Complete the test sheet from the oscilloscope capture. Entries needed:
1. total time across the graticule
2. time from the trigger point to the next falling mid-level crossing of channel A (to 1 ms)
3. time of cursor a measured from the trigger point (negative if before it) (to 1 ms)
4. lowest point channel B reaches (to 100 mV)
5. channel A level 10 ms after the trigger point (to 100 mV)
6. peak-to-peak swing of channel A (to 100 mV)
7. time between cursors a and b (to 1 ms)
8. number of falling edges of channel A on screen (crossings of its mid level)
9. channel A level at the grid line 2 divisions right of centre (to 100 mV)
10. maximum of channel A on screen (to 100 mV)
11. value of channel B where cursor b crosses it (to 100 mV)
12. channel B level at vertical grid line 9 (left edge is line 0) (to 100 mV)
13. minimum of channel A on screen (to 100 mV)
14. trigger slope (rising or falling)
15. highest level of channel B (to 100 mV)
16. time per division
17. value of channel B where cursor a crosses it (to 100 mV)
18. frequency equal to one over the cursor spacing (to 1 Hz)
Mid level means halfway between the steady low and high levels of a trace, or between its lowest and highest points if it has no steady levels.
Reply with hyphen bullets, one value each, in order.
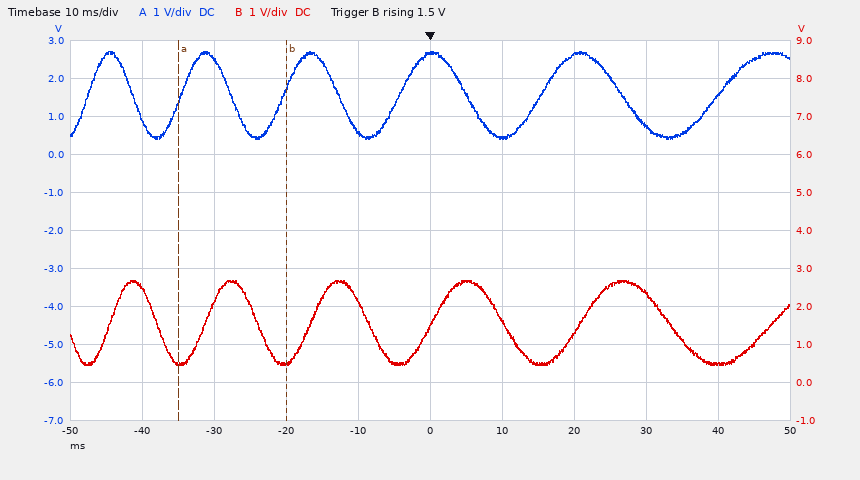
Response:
- 100 ms
- 5 ms
- -35 ms
- 400 mV
- 400 mV
- 2.3 V
- 15 ms
- 5
- 2.6 V
- 2.7 V
- 500 mV
- 500 mV
- 400 mV
- rising
- 2.7 V
- 10 ms
- 500 mV
- 67 Hz
